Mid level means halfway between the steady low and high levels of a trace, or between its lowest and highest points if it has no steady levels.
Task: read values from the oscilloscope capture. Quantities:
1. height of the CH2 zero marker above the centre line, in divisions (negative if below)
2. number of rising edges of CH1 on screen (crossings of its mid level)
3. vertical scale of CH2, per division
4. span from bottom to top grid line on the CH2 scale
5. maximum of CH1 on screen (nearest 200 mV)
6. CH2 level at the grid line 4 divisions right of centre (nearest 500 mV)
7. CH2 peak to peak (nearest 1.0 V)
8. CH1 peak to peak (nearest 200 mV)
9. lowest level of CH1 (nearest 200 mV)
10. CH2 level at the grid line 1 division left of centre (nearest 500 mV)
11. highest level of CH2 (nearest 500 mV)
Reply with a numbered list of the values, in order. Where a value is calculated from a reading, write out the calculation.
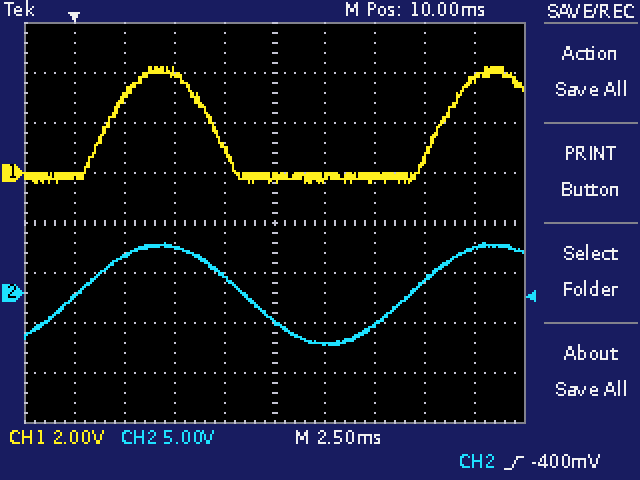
1. -1.4 div
2. 2
3. 5 V
4. 40 V
5. 4.2 V
6. 4.5 V
7. 10.0 V
8. 4.2 V − (-400 mV) = 4.6 V
9. -400 mV
10. 1.5 V
11. 5.0 V
